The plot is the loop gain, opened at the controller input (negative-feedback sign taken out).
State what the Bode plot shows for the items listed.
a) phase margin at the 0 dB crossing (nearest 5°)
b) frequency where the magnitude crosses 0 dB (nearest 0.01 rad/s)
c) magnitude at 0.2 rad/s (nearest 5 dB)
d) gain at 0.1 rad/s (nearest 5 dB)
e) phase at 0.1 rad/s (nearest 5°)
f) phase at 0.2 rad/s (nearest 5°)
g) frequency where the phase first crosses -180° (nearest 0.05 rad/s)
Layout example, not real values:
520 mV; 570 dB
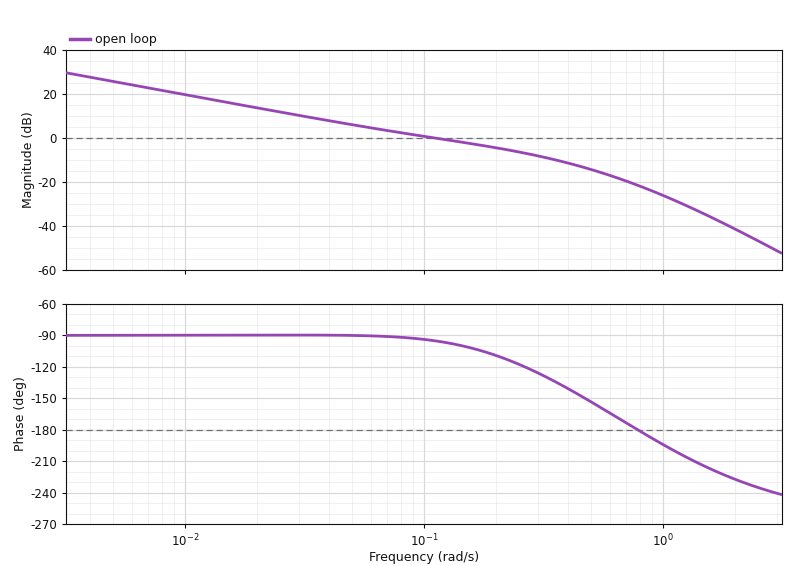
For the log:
85°; 0.11 rad/s; -5 dB; 0 dB; -95°; -110°; 0.80 rad/s
